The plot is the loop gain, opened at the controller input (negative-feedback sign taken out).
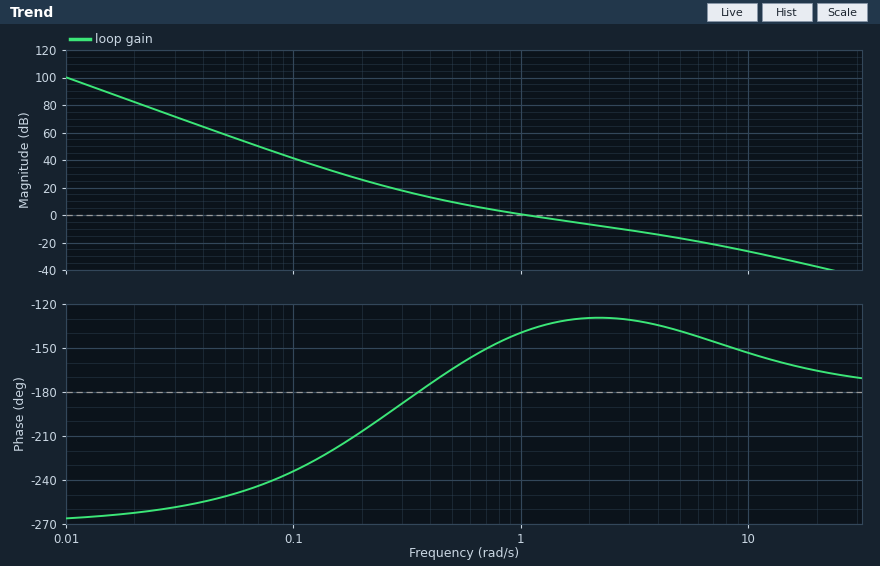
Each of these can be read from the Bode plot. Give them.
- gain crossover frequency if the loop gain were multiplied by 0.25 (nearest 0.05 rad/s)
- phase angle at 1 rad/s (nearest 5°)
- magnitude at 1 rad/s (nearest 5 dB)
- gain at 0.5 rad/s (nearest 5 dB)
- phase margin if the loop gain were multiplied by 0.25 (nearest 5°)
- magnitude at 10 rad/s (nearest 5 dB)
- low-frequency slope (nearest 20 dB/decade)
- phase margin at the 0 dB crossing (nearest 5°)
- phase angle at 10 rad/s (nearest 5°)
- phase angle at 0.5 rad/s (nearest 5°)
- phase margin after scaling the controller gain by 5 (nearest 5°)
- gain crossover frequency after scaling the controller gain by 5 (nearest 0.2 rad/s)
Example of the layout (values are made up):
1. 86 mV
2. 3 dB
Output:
1. 0.40 rad/s
2. -140°
3. 0 dB
4. 10 dB
5. 10°
6. -25 dB
7. -60 dB/decade
8. 40°
9. -155°
10. -165°
11. 45°
12. 4.0 rad/s
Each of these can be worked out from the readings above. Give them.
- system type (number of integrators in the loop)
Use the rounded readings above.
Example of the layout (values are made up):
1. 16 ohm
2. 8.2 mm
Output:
1. 3
